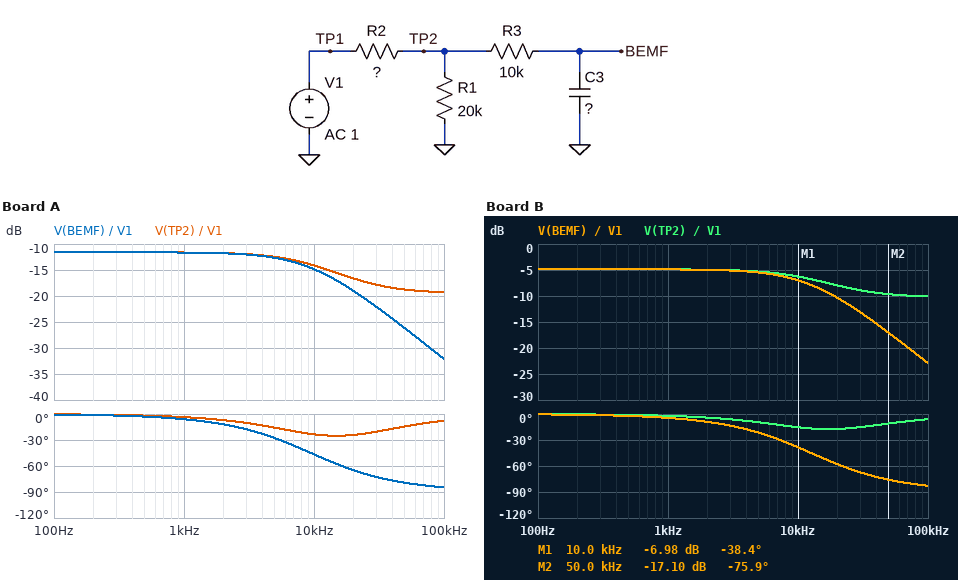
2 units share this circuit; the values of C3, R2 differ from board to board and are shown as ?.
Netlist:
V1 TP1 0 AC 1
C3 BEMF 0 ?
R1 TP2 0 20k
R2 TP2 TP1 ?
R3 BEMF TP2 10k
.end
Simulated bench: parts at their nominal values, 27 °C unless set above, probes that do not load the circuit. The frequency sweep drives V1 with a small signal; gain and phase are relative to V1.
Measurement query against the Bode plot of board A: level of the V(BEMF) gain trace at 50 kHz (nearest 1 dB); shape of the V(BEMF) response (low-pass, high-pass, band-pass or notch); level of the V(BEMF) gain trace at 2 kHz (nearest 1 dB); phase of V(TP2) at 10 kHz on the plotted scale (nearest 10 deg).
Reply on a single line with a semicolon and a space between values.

-26 dB; low-pass; -12 dB; -20 deg
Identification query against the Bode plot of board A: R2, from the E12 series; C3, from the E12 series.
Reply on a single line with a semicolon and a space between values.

56 kΩ; 680 pF
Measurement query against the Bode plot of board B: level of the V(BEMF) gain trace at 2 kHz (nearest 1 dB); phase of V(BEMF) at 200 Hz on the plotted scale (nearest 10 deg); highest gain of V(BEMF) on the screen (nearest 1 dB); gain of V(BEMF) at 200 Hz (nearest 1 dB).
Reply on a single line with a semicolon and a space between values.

-5 dB; 0 deg; -5 dB; -5 dB
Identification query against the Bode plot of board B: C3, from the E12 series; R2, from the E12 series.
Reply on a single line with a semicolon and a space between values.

680 pF; 15 kΩ
